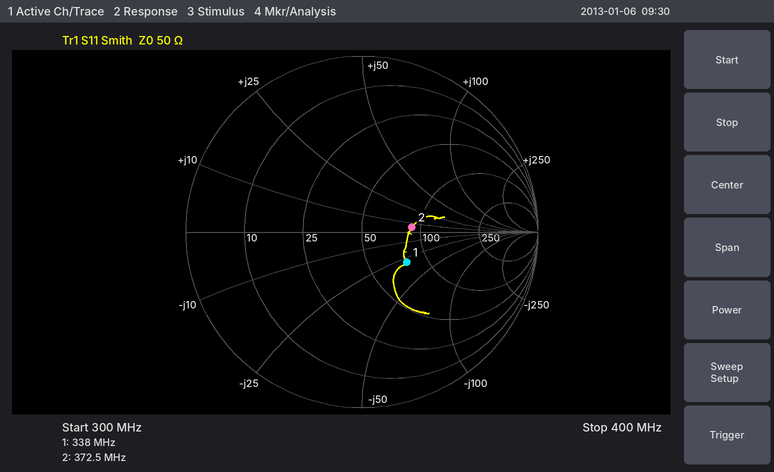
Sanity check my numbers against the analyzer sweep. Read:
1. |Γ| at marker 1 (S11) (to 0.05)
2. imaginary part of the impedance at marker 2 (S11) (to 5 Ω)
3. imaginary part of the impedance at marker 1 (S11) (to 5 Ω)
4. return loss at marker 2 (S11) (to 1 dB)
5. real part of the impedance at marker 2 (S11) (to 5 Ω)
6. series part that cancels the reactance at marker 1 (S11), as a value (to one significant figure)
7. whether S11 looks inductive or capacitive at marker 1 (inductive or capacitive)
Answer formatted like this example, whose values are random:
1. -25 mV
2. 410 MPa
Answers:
1. 0.30
2. +5 Ω
3. -30 Ω
4. 11 dB
5. 90 Ω
6. 10 nH
7. capacitive
